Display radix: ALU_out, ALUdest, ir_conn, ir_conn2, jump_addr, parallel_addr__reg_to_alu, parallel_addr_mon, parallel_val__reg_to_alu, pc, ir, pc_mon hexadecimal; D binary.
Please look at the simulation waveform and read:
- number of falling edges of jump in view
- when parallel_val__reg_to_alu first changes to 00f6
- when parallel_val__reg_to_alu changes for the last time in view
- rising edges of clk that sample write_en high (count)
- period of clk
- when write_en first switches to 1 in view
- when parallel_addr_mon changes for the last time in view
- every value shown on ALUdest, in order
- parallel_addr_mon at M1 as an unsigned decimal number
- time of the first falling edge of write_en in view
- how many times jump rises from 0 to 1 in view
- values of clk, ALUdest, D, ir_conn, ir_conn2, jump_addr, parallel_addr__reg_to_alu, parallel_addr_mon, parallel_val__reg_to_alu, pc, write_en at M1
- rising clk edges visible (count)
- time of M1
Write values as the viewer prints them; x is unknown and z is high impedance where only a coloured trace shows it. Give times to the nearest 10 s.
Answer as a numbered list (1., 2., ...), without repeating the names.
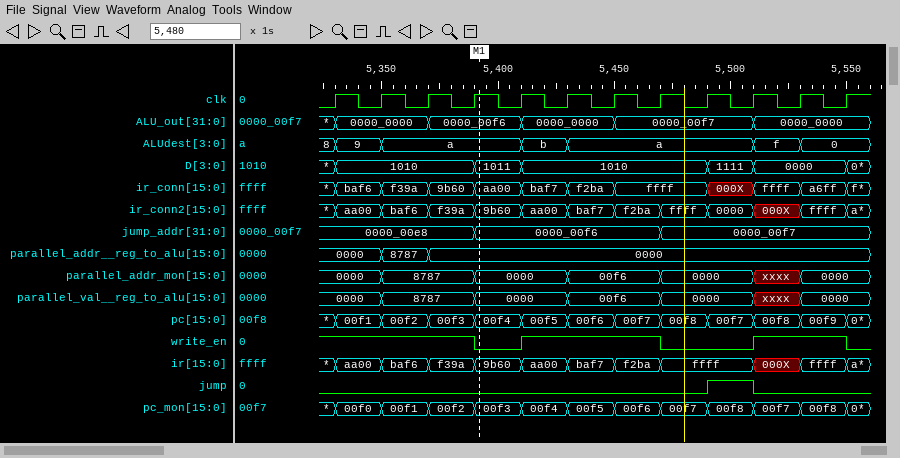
1. 1
2. 5430 s
3. 5530 s
4. 9
5. 20 s
6. 5410 s
7. 5530 s
8. 8, 9, a, b, a, f, 0
9. 0
10. 5390 s
11. 1
12. clk=1, ALUdest=a, D=1011, ir_conn=aa00, ir_conn2=9b60, jump_addr=0000_00f6, parallel_addr__reg_to_alu=0000, parallel_addr_mon=0000, parallel_val__reg_to_alu=0000, pc=00f4, write_en=0
13. 12
14. 5390 s
